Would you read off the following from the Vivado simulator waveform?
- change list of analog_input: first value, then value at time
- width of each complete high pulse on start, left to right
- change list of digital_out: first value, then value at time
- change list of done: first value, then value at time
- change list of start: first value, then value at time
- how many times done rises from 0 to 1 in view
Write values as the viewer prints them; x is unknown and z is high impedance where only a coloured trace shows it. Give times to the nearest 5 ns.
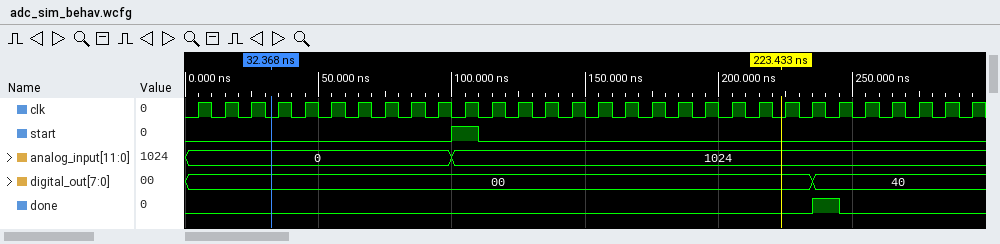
0, 1024 at 100 ns
10 ns
00, 40 at 235 ns
0, 1 at 235 ns, 0 at 245 ns
0, 1 at 100 ns, 0 at 110 ns
1
